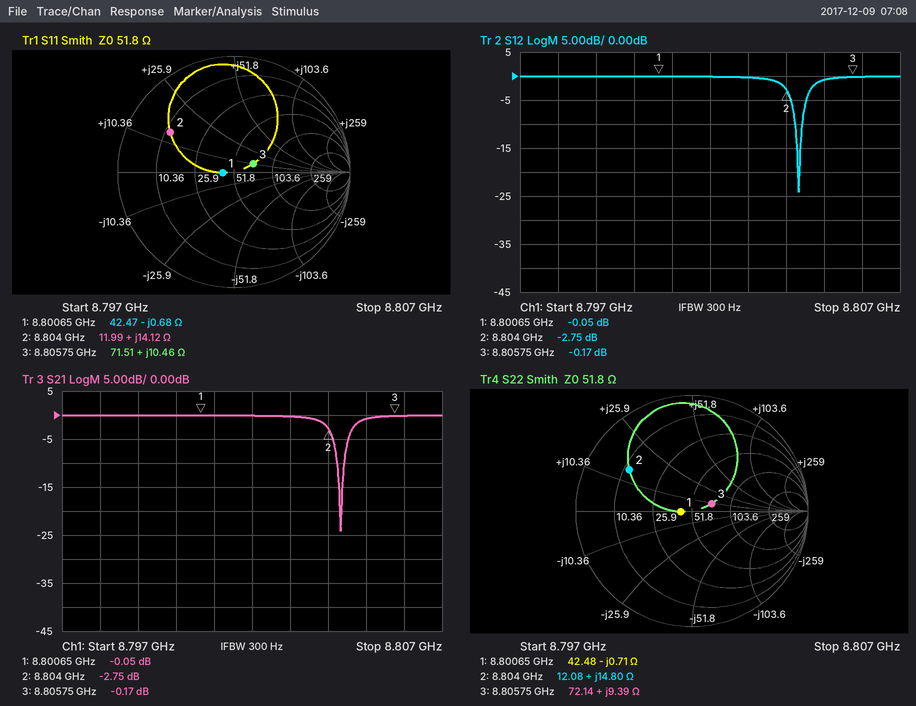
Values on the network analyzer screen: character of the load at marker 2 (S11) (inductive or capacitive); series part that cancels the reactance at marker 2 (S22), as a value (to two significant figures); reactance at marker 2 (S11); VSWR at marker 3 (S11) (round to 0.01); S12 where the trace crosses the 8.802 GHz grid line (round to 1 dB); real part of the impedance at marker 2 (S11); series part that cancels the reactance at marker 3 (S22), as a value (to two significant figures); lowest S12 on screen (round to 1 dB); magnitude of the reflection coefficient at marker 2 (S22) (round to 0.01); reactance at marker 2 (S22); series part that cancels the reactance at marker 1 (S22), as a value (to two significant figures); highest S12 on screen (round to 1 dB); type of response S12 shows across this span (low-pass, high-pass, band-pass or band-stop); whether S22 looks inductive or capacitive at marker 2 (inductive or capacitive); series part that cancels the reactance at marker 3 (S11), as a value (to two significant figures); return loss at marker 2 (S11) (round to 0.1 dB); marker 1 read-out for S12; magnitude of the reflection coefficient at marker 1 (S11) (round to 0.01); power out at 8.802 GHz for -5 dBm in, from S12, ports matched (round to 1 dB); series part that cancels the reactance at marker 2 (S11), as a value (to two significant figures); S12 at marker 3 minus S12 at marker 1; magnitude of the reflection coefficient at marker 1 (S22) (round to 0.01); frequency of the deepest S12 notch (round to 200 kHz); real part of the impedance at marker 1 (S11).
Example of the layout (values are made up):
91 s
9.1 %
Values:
inductive
1.2 pF
+14.12 Ω
1.44
0 dB
11.99 Ω
1.9 pF
-24 dB
0.65
+14.80 Ω
13 pH
0 dB
band-stop
inductive
1.7 pF
3.8 dB
-0.05 dB
0.10
-5 dBm
1.3 pF
-0.12 dB
0.10
8.8044 GHz
42.47 Ω
